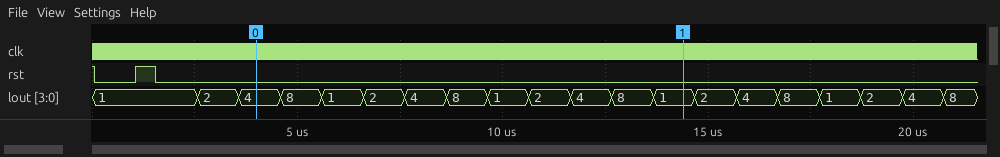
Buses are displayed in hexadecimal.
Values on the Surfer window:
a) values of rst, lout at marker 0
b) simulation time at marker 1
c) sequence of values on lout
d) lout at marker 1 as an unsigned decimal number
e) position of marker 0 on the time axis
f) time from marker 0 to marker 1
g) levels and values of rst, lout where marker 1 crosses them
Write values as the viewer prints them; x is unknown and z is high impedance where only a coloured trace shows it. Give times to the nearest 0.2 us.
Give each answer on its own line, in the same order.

rst=0, lout=4
14.4 us
1, 2, 4, 8, 1, 2, 4, 8, 1, 2, 4, 8, 1, 2, 4, 8, 1, 2, 4, 8
1
4 us
10.4 us
rst=0, lout=1
